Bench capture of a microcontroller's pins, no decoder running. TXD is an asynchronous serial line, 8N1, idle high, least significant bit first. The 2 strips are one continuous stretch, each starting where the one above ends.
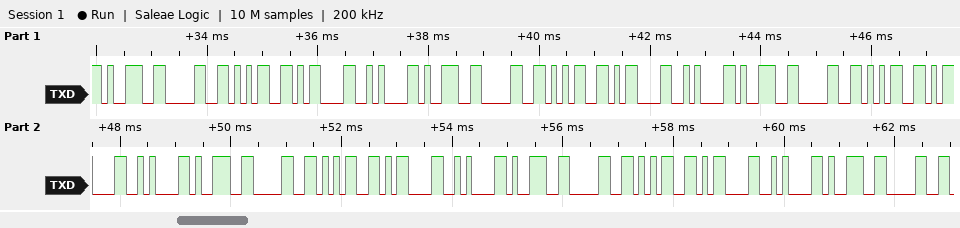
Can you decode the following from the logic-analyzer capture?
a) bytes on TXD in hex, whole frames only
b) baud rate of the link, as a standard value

39 30 35 0D 0A 39 30 35 0D 0A 39 30 35 0D 0A 39 30 35 0D 0A 39 30 35 0D 0A 39 30
9600 baud
